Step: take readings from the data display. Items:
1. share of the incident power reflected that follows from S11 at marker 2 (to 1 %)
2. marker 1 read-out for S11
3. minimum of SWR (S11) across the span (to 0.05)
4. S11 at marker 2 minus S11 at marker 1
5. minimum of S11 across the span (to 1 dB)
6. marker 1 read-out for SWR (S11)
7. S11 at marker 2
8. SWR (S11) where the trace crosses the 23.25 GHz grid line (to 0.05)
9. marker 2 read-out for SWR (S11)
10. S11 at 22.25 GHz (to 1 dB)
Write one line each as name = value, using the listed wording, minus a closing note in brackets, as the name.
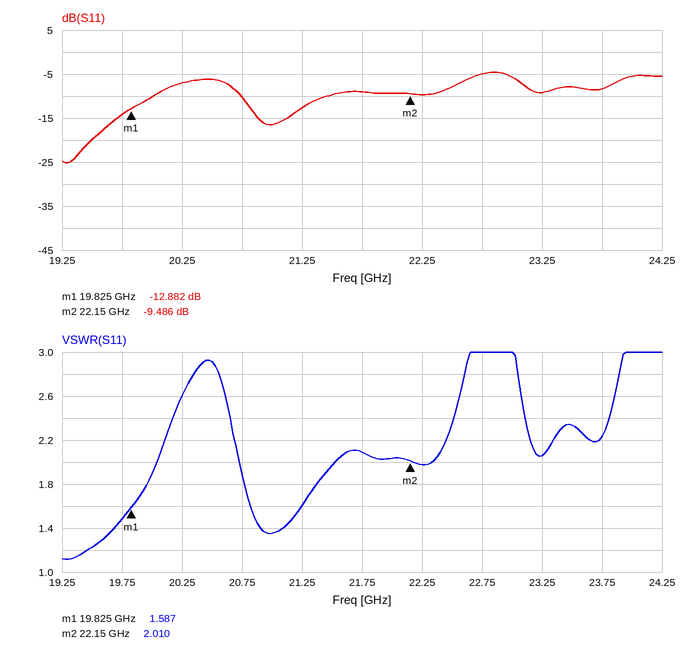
share of the incident power reflected that follows from S11 at marker 2 = 11 %
marker 1 read-out for S11 = -12.882 dB
minimum of SWR (S11) across the span = 1.10
S11 at marker 2 minus S11 at marker 1 = 3.396 dB
minimum of S11 across the span = -25 dB
marker 1 read-out for SWR = 1.587
S11 at marker 2 = -9.486 dB
SWR (S11) where the trace crosses the 23.25 GHz grid line = 2.05
marker 2 read-out for SWR = 2.010
S11 at 22.25 GHz = -10 dB
